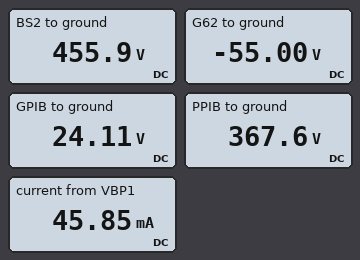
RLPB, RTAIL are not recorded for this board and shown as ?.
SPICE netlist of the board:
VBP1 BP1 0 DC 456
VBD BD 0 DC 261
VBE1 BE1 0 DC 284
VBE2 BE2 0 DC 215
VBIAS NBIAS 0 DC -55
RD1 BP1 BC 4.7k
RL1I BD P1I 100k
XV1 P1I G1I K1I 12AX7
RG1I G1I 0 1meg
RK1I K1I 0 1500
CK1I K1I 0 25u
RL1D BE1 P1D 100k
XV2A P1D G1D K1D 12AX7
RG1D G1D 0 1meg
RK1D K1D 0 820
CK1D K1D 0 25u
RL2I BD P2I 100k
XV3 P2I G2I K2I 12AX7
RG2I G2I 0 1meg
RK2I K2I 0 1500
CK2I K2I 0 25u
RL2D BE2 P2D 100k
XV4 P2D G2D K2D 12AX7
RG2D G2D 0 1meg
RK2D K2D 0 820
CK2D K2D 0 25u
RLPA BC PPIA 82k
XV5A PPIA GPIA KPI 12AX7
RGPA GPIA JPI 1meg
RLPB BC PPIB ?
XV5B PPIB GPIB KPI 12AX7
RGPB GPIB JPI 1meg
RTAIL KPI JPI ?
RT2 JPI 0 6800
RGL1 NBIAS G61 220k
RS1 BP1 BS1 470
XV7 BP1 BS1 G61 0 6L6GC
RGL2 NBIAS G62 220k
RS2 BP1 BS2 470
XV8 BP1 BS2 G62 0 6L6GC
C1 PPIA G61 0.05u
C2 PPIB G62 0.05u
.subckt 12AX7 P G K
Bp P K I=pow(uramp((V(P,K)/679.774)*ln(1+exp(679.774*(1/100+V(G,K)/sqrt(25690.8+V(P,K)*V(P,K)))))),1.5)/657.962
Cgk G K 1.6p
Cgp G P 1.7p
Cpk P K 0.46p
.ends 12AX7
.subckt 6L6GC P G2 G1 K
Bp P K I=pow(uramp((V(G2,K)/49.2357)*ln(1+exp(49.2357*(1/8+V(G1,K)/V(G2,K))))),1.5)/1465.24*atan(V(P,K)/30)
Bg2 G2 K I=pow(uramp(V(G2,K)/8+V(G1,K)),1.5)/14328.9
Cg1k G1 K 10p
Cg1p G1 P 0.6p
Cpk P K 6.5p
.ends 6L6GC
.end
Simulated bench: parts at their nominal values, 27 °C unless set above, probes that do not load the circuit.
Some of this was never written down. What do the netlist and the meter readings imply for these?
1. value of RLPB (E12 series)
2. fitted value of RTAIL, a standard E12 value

33 kΩ
680 Ω
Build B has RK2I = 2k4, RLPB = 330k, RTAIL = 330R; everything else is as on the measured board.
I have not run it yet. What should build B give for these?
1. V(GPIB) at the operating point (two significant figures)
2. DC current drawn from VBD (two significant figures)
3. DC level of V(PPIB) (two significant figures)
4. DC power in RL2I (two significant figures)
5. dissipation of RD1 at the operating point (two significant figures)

22 V
1.6 mA
160 V
51 mW
49 mW
